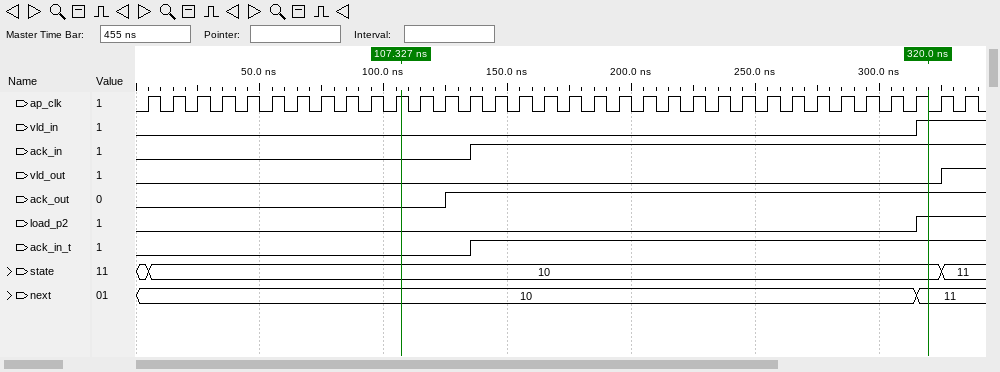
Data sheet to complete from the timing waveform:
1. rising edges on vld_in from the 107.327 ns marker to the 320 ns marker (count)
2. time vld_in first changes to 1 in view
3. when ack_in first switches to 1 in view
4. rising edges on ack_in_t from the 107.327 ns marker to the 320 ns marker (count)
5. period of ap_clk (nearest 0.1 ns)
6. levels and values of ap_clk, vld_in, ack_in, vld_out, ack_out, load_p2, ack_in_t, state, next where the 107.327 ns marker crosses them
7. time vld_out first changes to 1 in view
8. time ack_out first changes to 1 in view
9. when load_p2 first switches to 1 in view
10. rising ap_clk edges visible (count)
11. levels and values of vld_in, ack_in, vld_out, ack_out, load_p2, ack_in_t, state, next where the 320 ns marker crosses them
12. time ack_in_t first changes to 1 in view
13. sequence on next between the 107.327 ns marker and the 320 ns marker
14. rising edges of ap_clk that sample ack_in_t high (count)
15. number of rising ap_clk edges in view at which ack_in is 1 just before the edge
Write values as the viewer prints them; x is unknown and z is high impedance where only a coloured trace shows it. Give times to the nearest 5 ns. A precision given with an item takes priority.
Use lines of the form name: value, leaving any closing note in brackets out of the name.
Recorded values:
rising edges on vld_in from the 107.327 ns marker to the 320 ns marker: 1
time vld_in first changes to 1 in view: 315 ns
when ack_in first switches to 1 in view: 135 ns
rising edges on ack_in_t from the 107.327 ns marker to the 320 ns marker: 1
period of ap_clk: 10 ns
levels and values of ap_clk, vld_in, ack_in, vld_out, ack_out, load_p2, ack_in_t, state, next where the 107.327 ns marker crosses them: ap_clk=1, vld_in=0, ack_in=0, vld_out=0, ack_out=0, load_p2=0, ack_in_t=0, state=10, next=10
time vld_out first changes to 1 in view: 325 ns
time ack_out first changes to 1 in view: 125 ns
when load_p2 first switches to 1 in view: 315 ns
rising ap_clk edges visible: 34
levels and values of vld_in, ack_in, vld_out, ack_out, load_p2, ack_in_t, state, next where the 320 ns marker crosses them: vld_in=1, ack_in=1, vld_out=0, ack_out=1, load_p2=1, ack_in_t=1, state=10, next=11
time ack_in_t first changes to 1 in view: 135 ns
sequence on next between the 107.327 ns marker and the 320 ns marker: 10, 11
rising edges of ap_clk that sample ack_in_t high: 20
number of rising ap_clk edges in view at which ack_in is 1 just before the edge: 20
